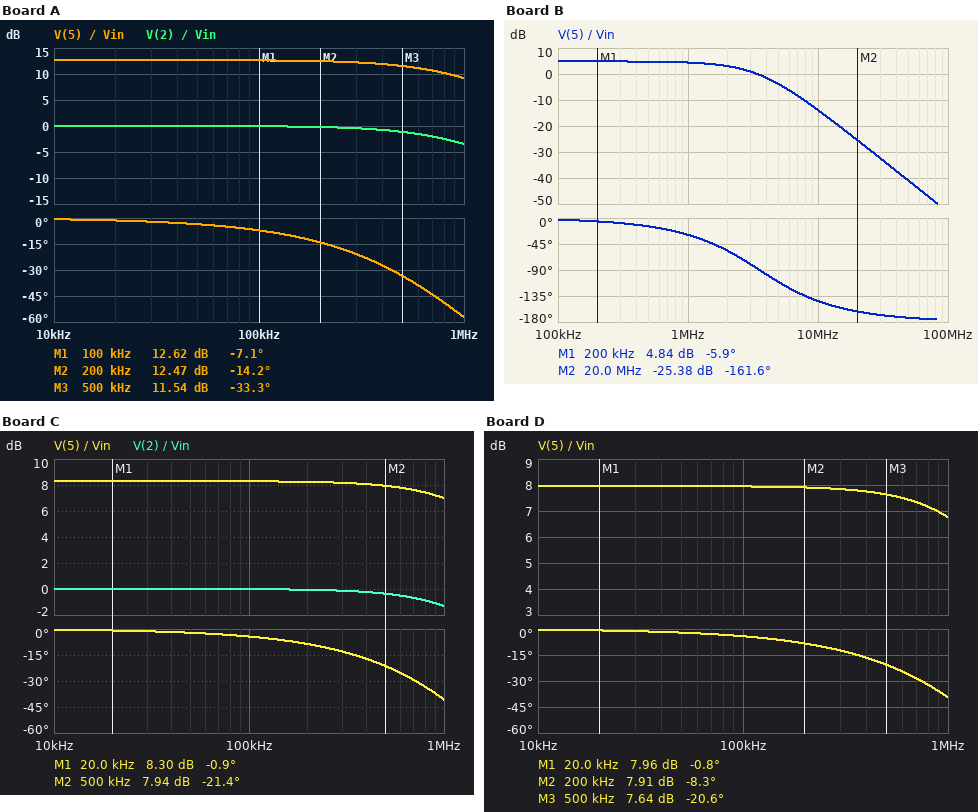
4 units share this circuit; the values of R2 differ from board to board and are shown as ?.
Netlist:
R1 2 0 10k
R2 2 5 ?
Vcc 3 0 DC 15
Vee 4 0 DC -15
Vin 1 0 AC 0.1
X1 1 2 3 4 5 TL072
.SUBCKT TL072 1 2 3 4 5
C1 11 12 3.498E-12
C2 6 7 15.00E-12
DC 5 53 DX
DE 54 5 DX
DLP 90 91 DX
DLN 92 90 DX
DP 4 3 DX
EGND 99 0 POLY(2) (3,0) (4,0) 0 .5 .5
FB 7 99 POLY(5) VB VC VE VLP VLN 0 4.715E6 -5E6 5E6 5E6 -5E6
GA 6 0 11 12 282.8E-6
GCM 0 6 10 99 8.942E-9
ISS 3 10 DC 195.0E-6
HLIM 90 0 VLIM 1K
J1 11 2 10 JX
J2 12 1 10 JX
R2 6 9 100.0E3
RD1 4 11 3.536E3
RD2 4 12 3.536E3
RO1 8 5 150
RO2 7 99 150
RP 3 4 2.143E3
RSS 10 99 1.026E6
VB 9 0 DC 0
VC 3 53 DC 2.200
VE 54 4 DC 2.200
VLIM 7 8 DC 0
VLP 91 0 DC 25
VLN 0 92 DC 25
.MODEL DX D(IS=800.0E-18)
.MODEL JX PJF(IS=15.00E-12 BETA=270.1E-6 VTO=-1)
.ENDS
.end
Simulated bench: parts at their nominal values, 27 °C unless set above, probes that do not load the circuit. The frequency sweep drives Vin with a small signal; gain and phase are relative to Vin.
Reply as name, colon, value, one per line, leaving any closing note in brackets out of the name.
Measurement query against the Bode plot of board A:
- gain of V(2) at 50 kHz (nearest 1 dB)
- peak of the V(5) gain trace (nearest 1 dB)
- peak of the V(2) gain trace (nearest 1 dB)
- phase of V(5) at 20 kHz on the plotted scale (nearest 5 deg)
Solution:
gain of V(2) at 50 kHz: 0 dB
peak of the V(5) gain trace: 13 dB
peak of the V(2) gain trace: 0 dB
phase of V(5) at 20 kHz on the plotted scale: 0 deg
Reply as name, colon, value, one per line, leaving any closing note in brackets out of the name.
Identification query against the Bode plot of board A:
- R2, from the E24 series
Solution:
R2, from the E24 series: 33 kΩ
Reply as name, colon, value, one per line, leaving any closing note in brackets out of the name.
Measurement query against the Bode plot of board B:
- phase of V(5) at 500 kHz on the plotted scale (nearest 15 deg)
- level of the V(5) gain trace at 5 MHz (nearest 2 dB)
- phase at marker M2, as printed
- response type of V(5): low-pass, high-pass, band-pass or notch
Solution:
phase of V(5) at 500 kHz on the plotted scale: -15 deg
level of the V(5) gain trace at 5 MHz: -4 dB
phase at marker M2, as printed: -161.6 deg
response type of V(5): low-pass, high-pass, band-pass or notch: low-pass
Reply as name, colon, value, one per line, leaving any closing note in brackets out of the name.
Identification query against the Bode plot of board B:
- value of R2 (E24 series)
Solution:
value of R2: 7.5 kΩ
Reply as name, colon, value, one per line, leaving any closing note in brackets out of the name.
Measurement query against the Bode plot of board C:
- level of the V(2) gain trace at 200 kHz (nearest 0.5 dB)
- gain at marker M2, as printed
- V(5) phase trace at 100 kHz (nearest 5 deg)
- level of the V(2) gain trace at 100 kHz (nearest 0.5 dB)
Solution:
level of the V(2) gain trace at 200 kHz: 0 dB
gain at marker M2, as printed: 7.94 dB
V(5) phase trace at 100 kHz: -5 deg
level of the V(2) gain trace at 100 kHz: 0 dB
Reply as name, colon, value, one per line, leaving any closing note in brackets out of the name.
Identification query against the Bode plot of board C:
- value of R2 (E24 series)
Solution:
value of R2: 16 kΩ
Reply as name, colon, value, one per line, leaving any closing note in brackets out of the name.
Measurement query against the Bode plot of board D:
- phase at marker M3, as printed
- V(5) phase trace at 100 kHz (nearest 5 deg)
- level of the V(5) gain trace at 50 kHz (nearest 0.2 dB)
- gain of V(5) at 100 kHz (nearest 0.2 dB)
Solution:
phase at marker M3, as printed: -20.6 deg
V(5) phase trace at 100 kHz: -5 deg
level of the V(5) gain trace at 50 kHz: 8.0 dB
gain of V(5) at 100 kHz: 8.0 dB
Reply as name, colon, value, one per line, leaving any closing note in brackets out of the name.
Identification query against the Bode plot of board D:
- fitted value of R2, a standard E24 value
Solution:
fitted value of R2, a standard E24 value: 15 kΩ
